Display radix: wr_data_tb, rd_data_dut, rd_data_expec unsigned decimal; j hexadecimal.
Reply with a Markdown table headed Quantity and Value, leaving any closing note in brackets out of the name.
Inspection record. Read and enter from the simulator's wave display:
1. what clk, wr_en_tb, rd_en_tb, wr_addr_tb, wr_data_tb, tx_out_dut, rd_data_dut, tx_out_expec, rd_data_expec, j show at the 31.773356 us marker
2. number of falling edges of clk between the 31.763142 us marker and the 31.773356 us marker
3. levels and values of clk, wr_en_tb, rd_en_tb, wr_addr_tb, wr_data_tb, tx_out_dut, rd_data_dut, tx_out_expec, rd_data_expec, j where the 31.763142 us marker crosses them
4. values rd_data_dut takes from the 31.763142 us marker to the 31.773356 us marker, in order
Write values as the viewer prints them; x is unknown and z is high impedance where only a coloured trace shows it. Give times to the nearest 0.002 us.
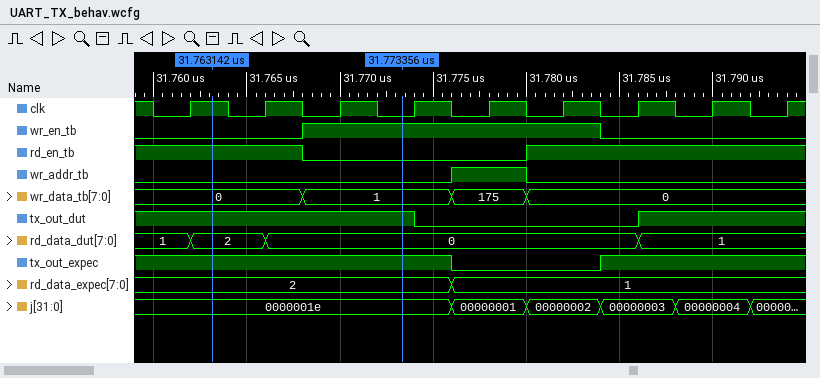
| Quantity | Value |
|---|---|
| what clk, wr_en_tb, rd_en_tb, wr_addr_tb, wr_data_tb, tx_out_dut, rd_data_dut, tx_out_expec, rd_data_expec, j show at the 31.773356 us marker | clk=0, wr_en_tb=1, rd_en_tb=0, wr_addr_tb=0, wr_data_tb=1, tx_out_dut=1, rd_data_dut=0, tx_out_expec=1, rd_data_expec=2, j=0000001e |
| number of falling edges of clk between the 31.763142 us marker and the 31.773356 us marker | 3 |
| levels and values of clk, wr_en_tb, rd_en_tb, wr_addr_tb, wr_data_tb, tx_out_dut, rd_data_dut, tx_out_expec, rd_data_expec, j where the 31.763142 us marker crosses them | clk=1, wr_en_tb=0, rd_en_tb=1, wr_addr_tb=0, wr_data_tb=0, tx_out_dut=1, rd_data_dut=2, tx_out_expec=1, rd_data_expec=2, j=0000001e |
| values rd_data_dut takes from the 31.763142 us marker to the 31.773356 us marker, in order | 2, 0 |
